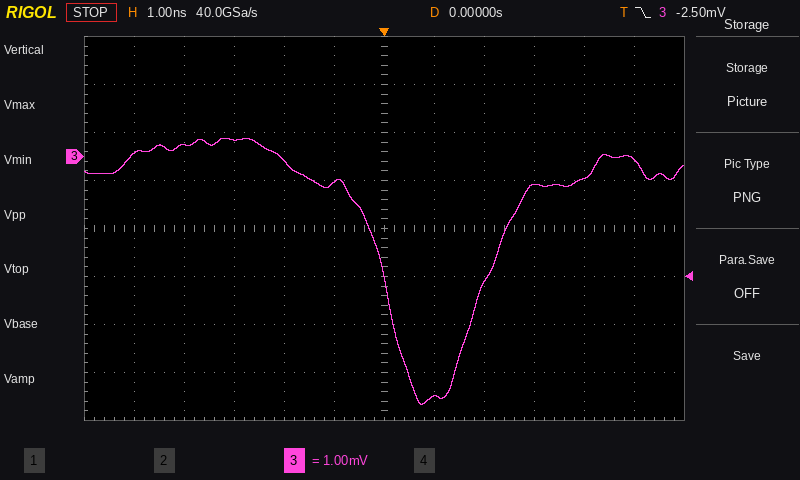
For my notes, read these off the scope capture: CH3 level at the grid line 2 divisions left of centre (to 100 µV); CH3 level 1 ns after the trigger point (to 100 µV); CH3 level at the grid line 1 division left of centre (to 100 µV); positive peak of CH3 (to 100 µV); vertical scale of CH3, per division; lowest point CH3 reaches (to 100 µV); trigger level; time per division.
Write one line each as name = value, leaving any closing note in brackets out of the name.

CH3 level at the grid line 2 divisions left of centre = -100 µV
CH3 level 1 ns after the trigger point = -5.0 mV
CH3 level at the grid line 1 division left of centre = -500 µV
positive peak of CH3 = 400 µV
vertical scale of CH3, per division = 1 mV
lowest point CH3 reaches = -5.2 mV
trigger level = -2.50 mV
time per division = 1 ns
